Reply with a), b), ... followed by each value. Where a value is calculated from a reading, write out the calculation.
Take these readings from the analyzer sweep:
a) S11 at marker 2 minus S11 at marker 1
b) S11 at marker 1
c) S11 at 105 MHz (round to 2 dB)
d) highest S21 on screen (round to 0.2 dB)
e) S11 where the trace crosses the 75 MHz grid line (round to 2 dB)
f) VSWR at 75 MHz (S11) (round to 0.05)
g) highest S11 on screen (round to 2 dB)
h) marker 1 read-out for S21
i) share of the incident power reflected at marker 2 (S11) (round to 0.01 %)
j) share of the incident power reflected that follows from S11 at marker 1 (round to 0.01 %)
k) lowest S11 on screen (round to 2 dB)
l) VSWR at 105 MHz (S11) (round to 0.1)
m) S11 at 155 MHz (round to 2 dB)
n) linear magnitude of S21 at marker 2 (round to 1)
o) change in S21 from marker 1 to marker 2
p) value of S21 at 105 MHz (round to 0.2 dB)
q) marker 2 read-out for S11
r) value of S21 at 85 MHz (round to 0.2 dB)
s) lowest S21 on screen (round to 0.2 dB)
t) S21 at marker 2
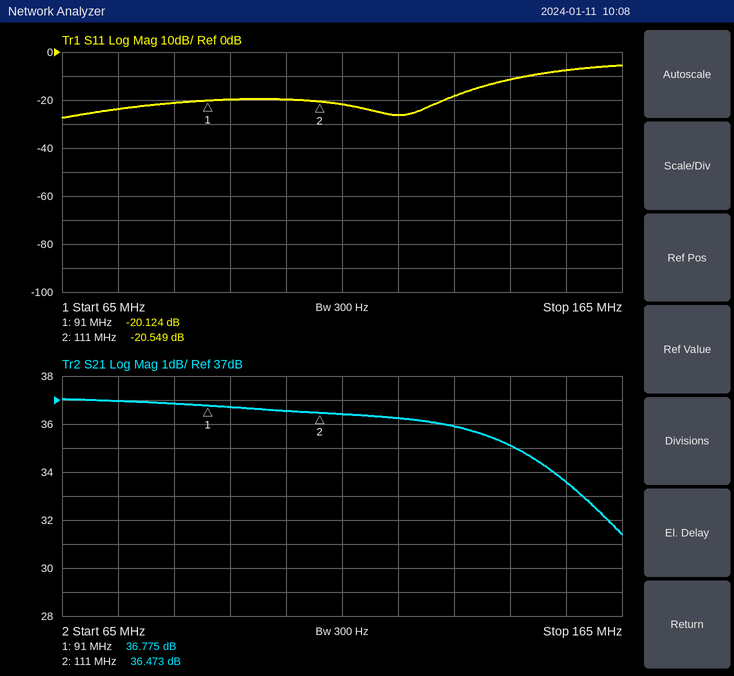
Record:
a) -20.549 − (-20.124) = -0.425 dB
b) -20.124 dB
c) -20 dB
d) 37.0 dB
e) -24 dB
f) |Γ| = 10^(-24/20) = 0.0631; VSWR = (1 + 0.0631)/(1 − 0.0631) ≈ 1.13, so 1.15 to the nearest 0.05
g) -6 dB
h) 36.775 dB
i) 10^(-20.549/10) ≈ 0.88 %
j) 10^(-20.124/10) ≈ 0.97 %
k) -28 dB
l) |Γ| = 10^(-20/20) = 0.1000; VSWR = (1 + 0.1000)/(1 − 0.1000) ≈ 1.2
m) -8 dB
n) 10^(36.473/20) ≈ 67
o) 36.473 − (36.775) = -0.302 dB
p) 36.6 dB
q) -20.549 dB
r) 36.8 dB
s) 31.4 dB
t) 36.473 dB
